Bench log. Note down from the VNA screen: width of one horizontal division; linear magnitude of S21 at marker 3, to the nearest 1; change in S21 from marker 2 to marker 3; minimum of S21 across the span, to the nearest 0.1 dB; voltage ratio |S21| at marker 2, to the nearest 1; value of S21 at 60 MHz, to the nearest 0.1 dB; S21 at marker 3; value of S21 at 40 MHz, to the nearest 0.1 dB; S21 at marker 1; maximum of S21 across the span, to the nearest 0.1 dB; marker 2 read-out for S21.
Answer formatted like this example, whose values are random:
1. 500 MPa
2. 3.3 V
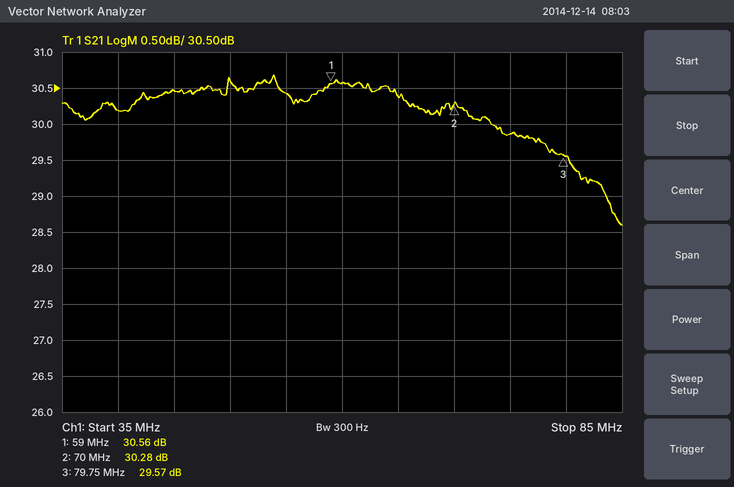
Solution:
1. 5 MHz
2. 30
3. -0.71 dB
4. 28.6 dB
5. 33
6. 30.6 dB
7. 29.57 dB
8. 30.2 dB
9. 30.56 dB
10. 30.7 dB
11. 30.28 dB
